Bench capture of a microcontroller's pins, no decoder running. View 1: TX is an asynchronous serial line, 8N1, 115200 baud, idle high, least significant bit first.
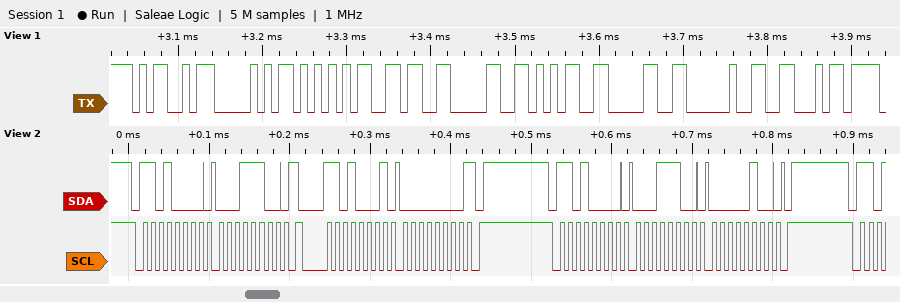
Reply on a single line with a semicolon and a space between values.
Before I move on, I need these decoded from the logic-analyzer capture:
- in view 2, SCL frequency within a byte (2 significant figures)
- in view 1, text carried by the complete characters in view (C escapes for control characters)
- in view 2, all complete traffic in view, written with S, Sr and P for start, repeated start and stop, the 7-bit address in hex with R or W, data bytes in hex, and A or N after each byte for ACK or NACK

100 kHz; "MPU6050 F"; S 68W A 1C A Sr 68R A 00 N P S 68W A 1C A 04 A P
